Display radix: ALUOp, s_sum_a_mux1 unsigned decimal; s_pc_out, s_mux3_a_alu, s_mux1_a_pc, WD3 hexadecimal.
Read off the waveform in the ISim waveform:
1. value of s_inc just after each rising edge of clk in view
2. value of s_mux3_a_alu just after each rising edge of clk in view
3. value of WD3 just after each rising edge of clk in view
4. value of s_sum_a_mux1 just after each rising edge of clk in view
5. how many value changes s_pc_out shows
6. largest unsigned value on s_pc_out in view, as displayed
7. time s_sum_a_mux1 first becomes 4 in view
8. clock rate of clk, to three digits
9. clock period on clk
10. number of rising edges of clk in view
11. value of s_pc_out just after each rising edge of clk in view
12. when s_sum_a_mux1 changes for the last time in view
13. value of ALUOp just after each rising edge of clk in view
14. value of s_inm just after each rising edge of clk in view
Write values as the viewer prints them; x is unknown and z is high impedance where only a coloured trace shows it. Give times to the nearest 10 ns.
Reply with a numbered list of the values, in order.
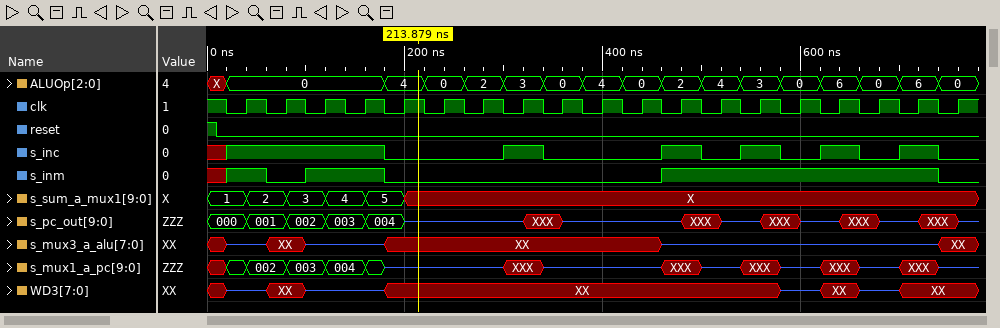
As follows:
1. 1 1 1 1 0 0 0 1 0 0 0 1 0 1 0 1 0 1 0
2. z, XX, z, z, XX, XX, XX, XX, XX, XX, XX, z, z, z, z, z, z, z, XX
3. z, XX, z, z, XX, XX, XX, XX, XX, XX, XX, XX, XX, XX, z, XX, z, XX, XX
4. 2, 3, 4, 5, X, X, X, X, X, X, X, X, X, X, X, X, X, X, X
5. 15
6. 004
7. 120 ns
8. 25.0 MHz
9. 40 ns
10. 19
11. 001, 002, 003, 004, z, z, z, XXX, z, z, z, XXX, z, XXX, z, XXX, z, XXX, z
12. 200 ns
13. 0, 0, 0, 0, 4, 0, 2, 3, 0, 4, 0, 2, 4, 3, 0, 6, 0, 6, 0
14. 1 0 1 1 0 0 0 0 0 0 0 1 1 1 1 1 1 1 0
